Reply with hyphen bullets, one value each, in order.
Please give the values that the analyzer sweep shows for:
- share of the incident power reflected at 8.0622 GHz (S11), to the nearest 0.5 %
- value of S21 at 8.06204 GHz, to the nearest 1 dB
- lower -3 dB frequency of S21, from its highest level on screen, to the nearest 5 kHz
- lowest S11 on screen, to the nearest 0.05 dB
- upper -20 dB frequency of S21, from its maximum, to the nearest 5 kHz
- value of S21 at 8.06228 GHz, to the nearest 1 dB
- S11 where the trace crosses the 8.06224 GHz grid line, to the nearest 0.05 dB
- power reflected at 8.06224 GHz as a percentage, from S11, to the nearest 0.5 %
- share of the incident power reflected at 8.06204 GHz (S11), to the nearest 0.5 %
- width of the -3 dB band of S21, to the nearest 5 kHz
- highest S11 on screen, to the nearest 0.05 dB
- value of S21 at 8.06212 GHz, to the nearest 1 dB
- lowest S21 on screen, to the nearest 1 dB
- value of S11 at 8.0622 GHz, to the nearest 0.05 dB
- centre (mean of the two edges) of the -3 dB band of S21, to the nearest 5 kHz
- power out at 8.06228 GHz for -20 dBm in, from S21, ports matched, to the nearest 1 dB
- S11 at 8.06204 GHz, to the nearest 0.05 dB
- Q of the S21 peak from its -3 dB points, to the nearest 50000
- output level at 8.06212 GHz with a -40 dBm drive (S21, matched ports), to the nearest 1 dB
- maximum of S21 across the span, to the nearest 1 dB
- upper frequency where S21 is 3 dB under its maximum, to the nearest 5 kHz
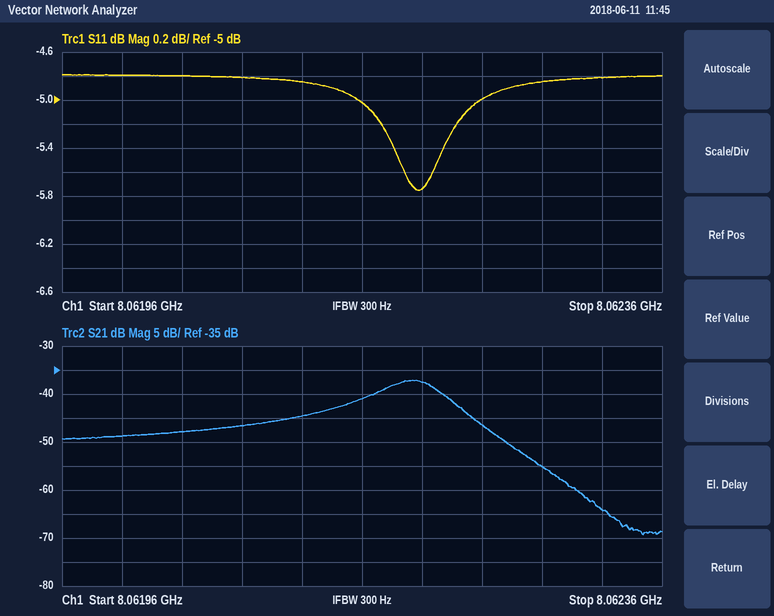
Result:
- 26.5 %
- -48 dB
- 8.062165 GHz
- -5.75 dB
- 8.062290 GHz
- -55 dB
- -5.00 dB
- 31.5 %
- 33.0 %
- 50 kHz
- -4.80 dB
- -45 dB
- -69 dB
- -5.75 dB
- 8.062190 GHz
- -75 dBm
- -4.80 dB
- 150000
- -85 dBm
- -37 dB
- 8.062215 GHz
